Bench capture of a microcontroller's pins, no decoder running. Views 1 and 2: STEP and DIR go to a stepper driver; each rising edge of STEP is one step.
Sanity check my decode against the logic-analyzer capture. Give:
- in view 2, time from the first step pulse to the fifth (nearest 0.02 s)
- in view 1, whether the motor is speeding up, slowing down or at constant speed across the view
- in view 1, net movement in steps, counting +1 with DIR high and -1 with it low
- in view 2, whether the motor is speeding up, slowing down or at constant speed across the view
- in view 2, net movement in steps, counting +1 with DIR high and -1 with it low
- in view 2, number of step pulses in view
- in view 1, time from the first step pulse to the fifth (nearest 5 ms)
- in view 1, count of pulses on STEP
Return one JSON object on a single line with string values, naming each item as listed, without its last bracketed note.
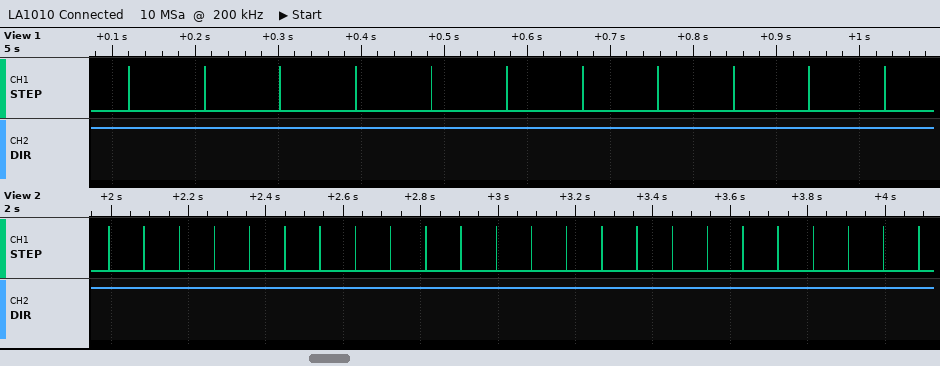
{"in view 2, time from the first step pulse to the fifth": "0.36 s", "in view 1, whether the motor is speeding up, slowing down or at constant speed across the view": "constant speed", "in view 1, net movement in steps, counting +1 with DIR high and -1 with it low": "+11", "in view 2, whether the motor is speeding up, slowing down or at constant speed across the view": "constant speed", "in view 2, net movement in steps, counting +1 with DIR high and -1 with it low": "+24", "in view 2, number of step pulses in view": "24", "in view 1, time from the first step pulse to the fifth": "365 ms", "in view 1, count of pulses on STEP": "11"}
